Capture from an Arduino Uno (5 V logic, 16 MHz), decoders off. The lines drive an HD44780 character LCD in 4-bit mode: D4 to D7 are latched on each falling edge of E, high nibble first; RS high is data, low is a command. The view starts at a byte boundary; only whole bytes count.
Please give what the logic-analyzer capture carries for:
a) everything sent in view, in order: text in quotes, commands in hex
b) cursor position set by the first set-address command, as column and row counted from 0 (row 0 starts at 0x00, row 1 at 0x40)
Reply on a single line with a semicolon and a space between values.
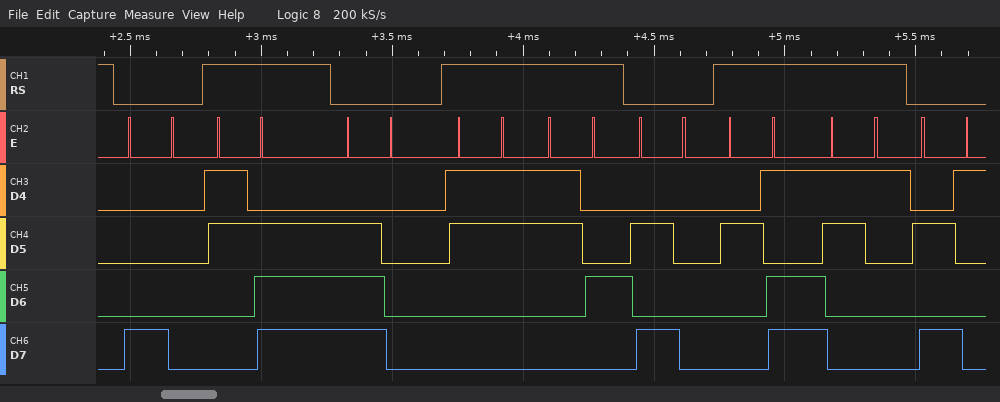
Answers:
0x80 ">" 0xE0 "34" 0xA0 "-1" 0xA1; column 0, row 0
